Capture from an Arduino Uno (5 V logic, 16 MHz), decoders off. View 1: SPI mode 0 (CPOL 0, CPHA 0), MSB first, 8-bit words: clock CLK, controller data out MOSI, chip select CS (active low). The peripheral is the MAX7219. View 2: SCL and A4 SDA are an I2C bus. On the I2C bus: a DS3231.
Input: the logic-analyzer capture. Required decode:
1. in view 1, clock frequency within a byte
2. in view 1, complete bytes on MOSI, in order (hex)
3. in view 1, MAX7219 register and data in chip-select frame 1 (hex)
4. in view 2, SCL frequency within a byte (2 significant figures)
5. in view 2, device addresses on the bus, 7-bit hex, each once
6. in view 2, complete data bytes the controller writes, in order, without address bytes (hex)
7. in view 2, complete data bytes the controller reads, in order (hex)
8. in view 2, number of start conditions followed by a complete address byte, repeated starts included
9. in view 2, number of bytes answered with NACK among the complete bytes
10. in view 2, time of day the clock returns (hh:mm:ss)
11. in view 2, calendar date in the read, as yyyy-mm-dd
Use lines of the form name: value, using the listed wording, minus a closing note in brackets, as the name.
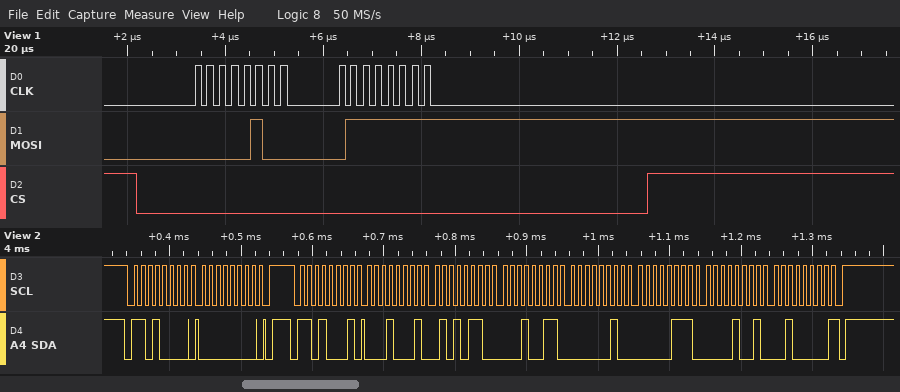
in view 1, clock frequency within a byte: 4 MHz
in view 1, complete bytes on MOSI, in order: 04 7F
in view 1, MAX7219 register and data in chip-select frame 1: register 0x4, data 0x7F
in view 2, SCL frequency within a byte: 100 kHz
in view 2, device addresses on the bus, 7-bit hex, each once: 0x68
in view 2, complete data bytes the controller writes, in order, without address bytes: 00
in view 2, complete data bytes the controller reads, in order: 11 56 13 02 07 09 20
in view 2, number of start conditions followed by a complete address byte, repeated starts included: 2
in view 2, number of bytes answered with NACK among the complete bytes: 1
in view 2, time of day the clock returns: 13:56:11
in view 2, calendar date in the read, as yyyy-mm-dd: 2020-09-07
